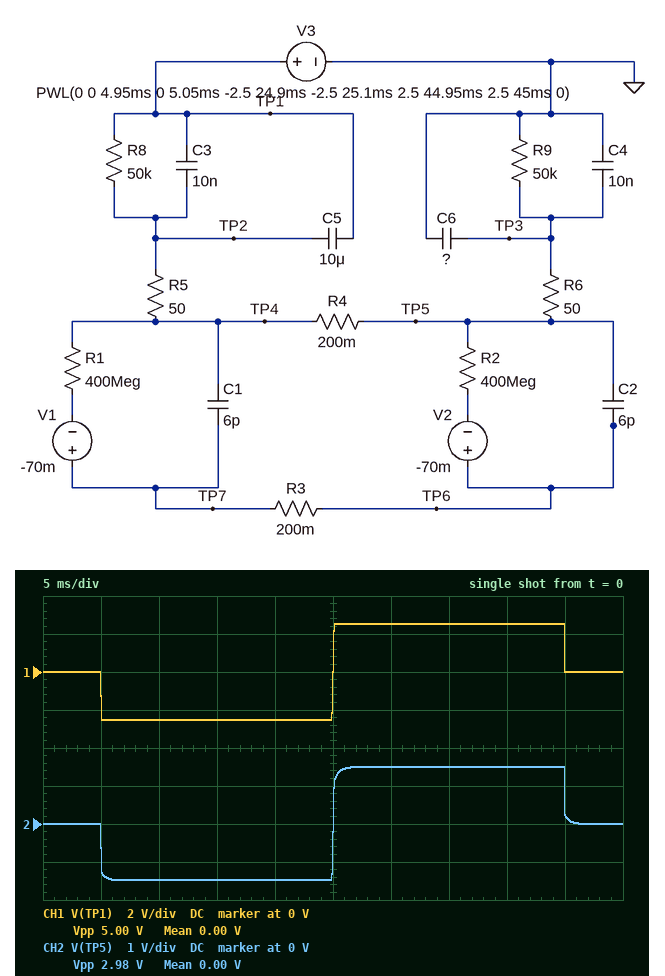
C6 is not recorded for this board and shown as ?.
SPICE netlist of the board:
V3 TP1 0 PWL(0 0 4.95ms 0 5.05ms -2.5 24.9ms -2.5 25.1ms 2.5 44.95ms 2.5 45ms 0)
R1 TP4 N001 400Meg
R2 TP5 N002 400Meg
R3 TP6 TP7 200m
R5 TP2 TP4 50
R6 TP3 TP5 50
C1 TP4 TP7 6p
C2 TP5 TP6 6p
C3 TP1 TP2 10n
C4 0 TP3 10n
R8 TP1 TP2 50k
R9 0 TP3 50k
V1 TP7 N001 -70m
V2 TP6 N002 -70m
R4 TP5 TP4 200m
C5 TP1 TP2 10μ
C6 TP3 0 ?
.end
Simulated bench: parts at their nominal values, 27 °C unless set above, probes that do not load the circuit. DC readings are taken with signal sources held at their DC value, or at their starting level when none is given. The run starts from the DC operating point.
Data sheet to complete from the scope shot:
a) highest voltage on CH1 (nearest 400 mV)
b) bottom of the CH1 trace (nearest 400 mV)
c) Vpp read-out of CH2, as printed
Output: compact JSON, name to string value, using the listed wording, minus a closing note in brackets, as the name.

{"highest voltage on CH1": "2.4 V", "bottom of the CH1 trace": "-2.4 V", "Vpp read-out of CH2, as printed": "2.98 V"}
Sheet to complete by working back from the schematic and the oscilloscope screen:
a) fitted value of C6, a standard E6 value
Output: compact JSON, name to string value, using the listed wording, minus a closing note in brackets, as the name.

{"fitted value of C6, a standard E6 value": "6.8 µF"}
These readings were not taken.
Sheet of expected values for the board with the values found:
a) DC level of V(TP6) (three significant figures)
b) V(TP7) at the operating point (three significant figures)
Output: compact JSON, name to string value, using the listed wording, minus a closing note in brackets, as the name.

{"DC level of V(TP6)": "-70.0 mV", "V(TP7) at the operating point": "-70.0 mV"}
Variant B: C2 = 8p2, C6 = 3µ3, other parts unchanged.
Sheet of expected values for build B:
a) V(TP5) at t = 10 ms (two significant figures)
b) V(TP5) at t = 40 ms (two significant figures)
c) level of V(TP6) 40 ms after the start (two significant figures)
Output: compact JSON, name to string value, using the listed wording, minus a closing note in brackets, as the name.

{"V(TP5) at t = 10 ms": "-1.9 V", "V(TP5) at t = 40 ms": "1.9 V", "level of V(TP6) 40 ms after the start": "1.8 V"}
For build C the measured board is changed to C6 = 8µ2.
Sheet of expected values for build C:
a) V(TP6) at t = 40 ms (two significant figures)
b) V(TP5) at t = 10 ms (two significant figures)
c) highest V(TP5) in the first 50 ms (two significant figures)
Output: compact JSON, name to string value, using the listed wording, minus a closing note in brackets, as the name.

{"V(TP6) at t = 40 ms": "1.3 V", "V(TP5) at t = 10 ms": "-1.4 V", "highest V(TP5) in the first 50 ms": "1.4 V"}
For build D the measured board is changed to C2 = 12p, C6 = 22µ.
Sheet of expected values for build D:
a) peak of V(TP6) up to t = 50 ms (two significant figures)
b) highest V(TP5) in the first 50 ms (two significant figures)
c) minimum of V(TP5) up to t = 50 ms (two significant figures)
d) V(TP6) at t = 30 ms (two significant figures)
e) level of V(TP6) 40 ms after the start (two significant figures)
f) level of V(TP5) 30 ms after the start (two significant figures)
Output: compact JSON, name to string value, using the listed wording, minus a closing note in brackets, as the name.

{"peak of V(TP6) up to t = 50 ms": "1.5 V", "highest V(TP5) in the first 50 ms": "1.6 V", "minimum of V(TP5) up to t = 50 ms": "-1.2 V", "V(TP6) at t = 30 ms": "700 mV", "level of V(TP6) 40 ms after the start": "710 mV", "level of V(TP5) 30 ms after the start": "770 mV"}
